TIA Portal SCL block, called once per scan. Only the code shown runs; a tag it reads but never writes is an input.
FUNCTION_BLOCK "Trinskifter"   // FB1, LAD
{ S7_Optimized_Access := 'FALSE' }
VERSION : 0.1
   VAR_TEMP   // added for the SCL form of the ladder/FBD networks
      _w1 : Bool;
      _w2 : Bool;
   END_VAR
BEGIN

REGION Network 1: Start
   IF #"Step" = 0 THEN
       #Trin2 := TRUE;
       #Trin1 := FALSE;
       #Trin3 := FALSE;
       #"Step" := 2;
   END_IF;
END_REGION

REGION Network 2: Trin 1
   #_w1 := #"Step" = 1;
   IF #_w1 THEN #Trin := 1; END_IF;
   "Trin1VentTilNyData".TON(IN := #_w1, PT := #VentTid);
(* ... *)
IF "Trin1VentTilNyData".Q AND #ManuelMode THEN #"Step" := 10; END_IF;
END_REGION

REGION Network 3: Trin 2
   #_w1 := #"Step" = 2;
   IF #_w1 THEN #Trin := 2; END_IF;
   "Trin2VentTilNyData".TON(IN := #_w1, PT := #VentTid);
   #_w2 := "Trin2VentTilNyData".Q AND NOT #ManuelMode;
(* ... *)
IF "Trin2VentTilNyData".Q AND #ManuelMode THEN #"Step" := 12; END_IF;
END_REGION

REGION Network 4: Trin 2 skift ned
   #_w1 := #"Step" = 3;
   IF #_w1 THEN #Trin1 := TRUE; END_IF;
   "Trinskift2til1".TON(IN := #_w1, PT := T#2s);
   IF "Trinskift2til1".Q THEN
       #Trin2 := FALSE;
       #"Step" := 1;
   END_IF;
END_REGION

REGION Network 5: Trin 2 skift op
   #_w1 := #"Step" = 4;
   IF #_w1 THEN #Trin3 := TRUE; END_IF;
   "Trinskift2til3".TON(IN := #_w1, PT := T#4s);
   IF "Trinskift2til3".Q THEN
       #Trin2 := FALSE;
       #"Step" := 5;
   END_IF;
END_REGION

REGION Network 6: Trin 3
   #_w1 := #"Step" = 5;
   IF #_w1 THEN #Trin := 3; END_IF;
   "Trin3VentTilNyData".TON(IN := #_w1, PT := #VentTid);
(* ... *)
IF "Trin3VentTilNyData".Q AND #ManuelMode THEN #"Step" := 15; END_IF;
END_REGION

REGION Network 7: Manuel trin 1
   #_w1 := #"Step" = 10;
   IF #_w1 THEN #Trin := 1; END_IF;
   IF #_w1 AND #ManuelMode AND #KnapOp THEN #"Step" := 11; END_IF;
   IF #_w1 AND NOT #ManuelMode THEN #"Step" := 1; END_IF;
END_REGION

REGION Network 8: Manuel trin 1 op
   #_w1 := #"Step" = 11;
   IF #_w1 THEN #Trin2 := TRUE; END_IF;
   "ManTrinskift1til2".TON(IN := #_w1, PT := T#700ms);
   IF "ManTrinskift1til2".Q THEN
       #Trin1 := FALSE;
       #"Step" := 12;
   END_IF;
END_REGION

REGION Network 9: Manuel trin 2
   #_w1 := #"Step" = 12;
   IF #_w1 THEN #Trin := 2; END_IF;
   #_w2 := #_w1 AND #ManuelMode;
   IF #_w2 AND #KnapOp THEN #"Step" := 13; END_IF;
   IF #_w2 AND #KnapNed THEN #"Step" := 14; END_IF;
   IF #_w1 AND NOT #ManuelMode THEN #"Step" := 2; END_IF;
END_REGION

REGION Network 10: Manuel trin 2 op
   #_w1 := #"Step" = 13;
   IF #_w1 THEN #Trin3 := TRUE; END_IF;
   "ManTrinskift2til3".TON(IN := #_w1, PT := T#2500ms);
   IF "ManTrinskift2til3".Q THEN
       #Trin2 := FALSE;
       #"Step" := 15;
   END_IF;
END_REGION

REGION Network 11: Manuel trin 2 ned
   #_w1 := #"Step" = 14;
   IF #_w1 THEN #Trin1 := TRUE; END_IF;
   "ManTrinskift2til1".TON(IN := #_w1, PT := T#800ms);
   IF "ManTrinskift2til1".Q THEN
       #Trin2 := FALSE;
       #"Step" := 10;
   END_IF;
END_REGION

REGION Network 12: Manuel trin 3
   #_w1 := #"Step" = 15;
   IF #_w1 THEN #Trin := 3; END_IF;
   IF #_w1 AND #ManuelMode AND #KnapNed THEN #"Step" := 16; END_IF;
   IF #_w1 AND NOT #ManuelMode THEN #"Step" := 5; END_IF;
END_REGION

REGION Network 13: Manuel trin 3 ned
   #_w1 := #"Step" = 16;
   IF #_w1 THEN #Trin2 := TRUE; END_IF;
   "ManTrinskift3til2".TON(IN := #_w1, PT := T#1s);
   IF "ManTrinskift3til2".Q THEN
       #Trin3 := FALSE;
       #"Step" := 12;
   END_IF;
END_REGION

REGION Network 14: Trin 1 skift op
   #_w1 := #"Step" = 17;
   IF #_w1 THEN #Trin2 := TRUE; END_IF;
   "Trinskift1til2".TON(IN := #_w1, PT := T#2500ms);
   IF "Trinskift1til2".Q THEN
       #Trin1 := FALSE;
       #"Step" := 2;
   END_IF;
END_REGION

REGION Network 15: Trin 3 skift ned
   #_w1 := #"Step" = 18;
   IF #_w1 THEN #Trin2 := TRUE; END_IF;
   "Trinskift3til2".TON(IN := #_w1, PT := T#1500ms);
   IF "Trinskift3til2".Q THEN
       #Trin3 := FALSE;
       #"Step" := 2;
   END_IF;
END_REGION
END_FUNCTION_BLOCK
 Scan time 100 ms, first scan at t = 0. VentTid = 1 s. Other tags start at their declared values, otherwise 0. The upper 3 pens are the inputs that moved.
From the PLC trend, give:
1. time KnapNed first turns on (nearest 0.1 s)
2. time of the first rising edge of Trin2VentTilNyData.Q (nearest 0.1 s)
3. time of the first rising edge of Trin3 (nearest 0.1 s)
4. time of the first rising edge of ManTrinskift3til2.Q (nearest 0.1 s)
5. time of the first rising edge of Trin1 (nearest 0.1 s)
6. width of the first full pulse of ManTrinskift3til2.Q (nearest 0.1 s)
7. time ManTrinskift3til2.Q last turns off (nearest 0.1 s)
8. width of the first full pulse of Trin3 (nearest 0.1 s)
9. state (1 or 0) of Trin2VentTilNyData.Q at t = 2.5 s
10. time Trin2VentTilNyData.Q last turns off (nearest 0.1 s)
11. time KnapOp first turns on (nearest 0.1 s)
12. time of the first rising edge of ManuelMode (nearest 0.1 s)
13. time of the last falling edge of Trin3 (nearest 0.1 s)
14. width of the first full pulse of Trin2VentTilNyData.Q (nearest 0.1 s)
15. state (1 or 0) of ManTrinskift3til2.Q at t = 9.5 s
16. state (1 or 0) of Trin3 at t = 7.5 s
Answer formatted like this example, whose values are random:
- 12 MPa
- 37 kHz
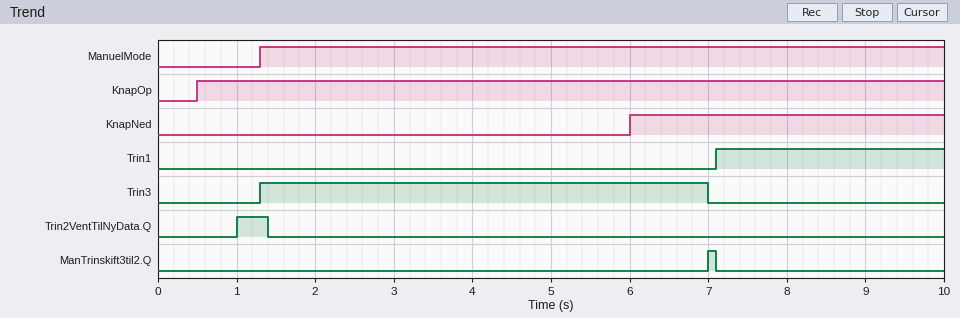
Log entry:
- 6.0 s
- 1.0 s
- 1.3 s
- 7.0 s
- 7.1 s
- 0.1 s
- 7.1 s
- 5.7 s
- 0
- 1.4 s
- 0.5 s
- 1.3 s
- 7.0 s
- 0.4 s
- 0
- 0
